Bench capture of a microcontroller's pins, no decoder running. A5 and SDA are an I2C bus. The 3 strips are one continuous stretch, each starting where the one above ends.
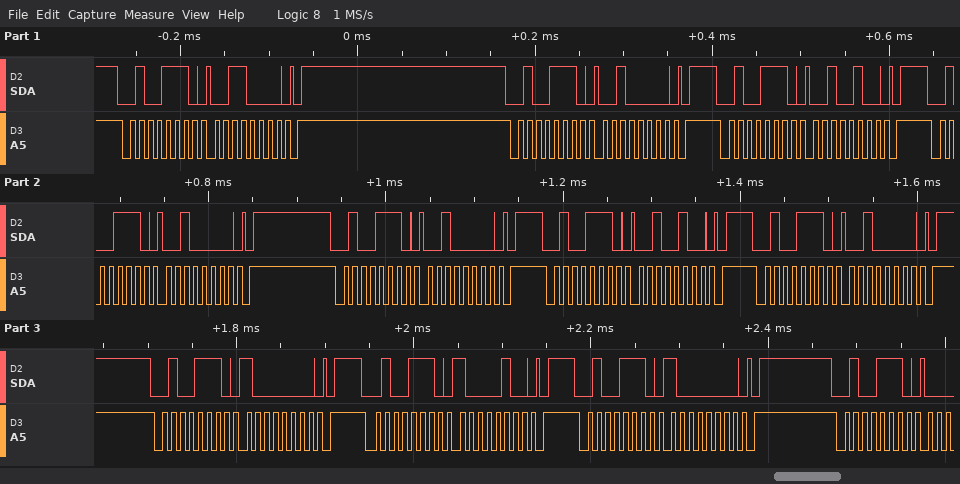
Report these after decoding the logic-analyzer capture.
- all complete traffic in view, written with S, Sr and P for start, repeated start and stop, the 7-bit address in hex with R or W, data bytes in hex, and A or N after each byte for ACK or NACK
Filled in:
S 27W A 30 A P S 27W A 20 A P S 27W A 24 A P S 27W A 20 A P S 27W A 20 A P S 27W A 24 A P S 27W A 20 A P S 27W A 80 A P S 27W A 84 A P S 27W A 80 A P S 27W A
